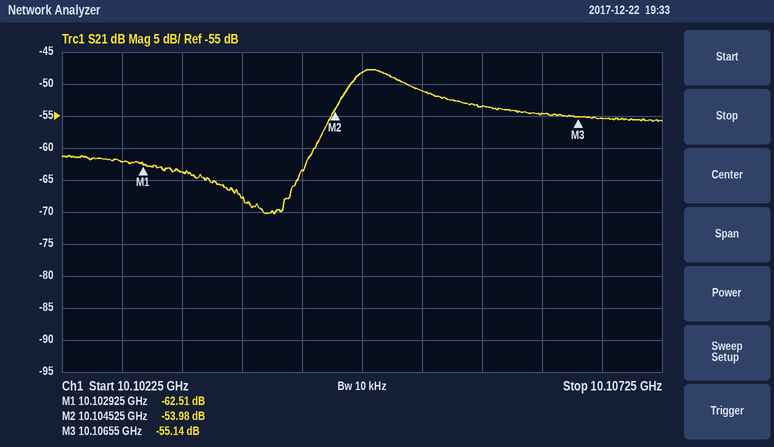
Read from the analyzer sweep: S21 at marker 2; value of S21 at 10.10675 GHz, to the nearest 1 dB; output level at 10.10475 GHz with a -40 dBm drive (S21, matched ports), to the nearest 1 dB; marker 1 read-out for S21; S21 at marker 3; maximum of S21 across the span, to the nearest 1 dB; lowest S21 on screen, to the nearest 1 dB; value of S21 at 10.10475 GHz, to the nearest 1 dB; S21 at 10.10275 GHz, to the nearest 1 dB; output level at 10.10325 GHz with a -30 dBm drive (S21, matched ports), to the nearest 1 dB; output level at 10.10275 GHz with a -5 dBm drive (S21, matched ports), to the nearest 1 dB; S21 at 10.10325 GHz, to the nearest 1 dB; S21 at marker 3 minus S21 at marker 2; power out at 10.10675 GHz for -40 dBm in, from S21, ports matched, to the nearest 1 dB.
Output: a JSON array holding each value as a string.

["-53.98 dB", "-55 dB", "-88 dBm", "-62.51 dB", "-55.14 dB", "-48 dB", "-70 dB", "-48 dB", "-62 dB", "-94 dBm", "-67 dBm", "-64 dB", "-1.16 dB", "-95 dBm"]
